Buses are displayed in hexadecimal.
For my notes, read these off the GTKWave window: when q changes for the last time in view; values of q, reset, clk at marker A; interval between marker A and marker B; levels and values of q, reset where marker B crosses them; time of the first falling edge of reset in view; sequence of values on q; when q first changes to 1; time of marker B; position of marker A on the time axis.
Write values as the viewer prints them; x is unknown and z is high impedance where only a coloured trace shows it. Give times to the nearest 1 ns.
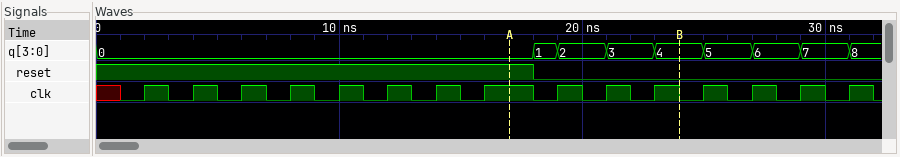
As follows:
31 ns
q=0, reset=1, clk=1
7 ns
q=4, reset=0
18 ns
0, 1, 2, 3, 4, 5, 6, 7, 8
18 ns
24 ns
17 ns
